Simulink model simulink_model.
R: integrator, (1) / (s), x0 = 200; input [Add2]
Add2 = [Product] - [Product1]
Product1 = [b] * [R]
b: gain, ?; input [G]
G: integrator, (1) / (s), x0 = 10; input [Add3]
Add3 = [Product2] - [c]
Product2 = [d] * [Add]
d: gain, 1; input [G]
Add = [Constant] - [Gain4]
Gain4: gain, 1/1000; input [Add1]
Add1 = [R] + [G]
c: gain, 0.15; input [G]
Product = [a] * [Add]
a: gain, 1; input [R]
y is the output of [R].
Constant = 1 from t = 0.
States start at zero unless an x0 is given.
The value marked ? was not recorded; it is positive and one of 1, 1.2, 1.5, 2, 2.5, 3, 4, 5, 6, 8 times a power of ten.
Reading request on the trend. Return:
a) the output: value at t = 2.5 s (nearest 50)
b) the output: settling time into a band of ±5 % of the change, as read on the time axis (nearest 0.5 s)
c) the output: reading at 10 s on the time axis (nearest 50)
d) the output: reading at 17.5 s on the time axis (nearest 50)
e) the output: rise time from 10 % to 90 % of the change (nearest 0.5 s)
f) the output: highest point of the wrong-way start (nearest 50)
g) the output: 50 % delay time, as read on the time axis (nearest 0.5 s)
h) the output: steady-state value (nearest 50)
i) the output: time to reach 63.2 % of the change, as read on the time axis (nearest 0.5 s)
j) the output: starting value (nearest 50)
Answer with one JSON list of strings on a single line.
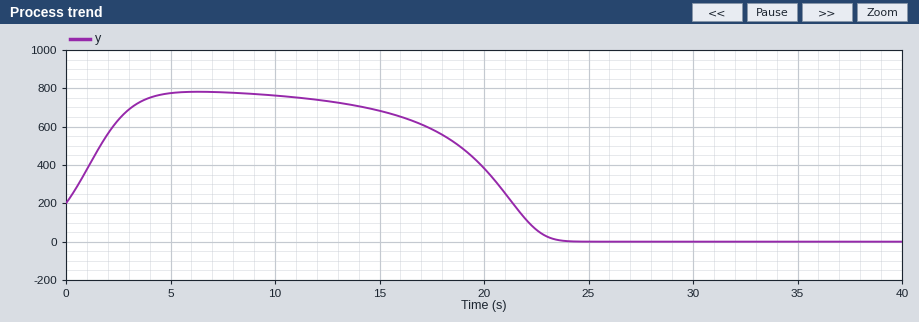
["650", "23.5 s", "750", "600", "1.5 s", "800", "22.0 s", "0", "22.5 s", "200"]
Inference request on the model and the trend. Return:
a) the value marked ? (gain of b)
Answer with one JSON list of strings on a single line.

["0.005"]
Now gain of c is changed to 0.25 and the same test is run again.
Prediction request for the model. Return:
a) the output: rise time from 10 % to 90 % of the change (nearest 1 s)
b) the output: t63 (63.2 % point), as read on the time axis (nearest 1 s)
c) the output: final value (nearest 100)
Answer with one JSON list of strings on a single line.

["8 s", "3 s", "1000"]
